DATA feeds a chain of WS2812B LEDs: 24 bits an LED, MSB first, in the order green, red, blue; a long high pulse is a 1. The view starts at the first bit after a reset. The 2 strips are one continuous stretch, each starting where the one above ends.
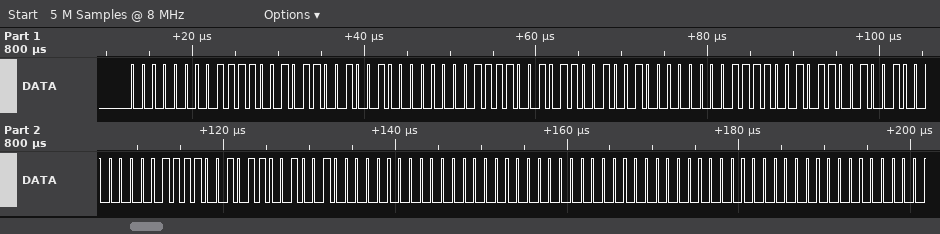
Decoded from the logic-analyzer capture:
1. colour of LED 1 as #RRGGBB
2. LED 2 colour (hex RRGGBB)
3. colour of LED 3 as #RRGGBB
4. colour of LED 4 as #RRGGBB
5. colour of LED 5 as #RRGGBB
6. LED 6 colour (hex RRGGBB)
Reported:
#F200C9
#F200C9
#F200C9
#F200C9
#000000
#000000
